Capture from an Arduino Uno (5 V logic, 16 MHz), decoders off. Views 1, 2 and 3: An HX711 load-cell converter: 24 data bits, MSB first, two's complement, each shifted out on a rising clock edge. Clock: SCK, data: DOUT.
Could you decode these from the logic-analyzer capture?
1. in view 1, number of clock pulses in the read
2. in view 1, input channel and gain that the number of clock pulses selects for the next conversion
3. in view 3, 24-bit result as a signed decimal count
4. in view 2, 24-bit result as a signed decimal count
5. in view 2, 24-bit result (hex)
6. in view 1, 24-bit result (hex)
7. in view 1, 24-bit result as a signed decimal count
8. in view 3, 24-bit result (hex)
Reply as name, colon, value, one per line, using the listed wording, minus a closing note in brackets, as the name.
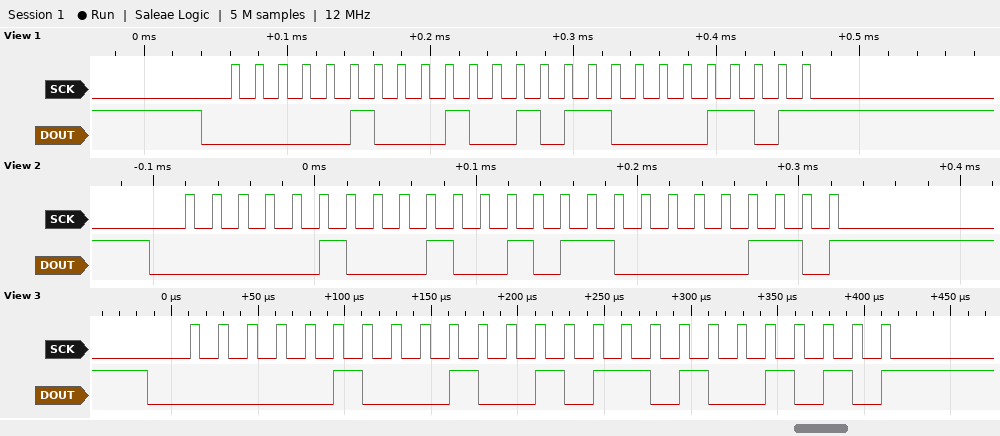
in view 1, number of clock pulses in the read: 25
in view 1, input channel and gain that the number of clock pulses selects for the next conversion: channel A, gain 128
in view 3, 24-bit result as a signed decimal count: 281418
in view 2, 24-bit result as a signed decimal count: 281350
in view 2, 24-bit result: 0x044B06
in view 1, 24-bit result: 0x044B0D
in view 1, 24-bit result as a signed decimal count: 281357
in view 3, 24-bit result: 0x044B4A
